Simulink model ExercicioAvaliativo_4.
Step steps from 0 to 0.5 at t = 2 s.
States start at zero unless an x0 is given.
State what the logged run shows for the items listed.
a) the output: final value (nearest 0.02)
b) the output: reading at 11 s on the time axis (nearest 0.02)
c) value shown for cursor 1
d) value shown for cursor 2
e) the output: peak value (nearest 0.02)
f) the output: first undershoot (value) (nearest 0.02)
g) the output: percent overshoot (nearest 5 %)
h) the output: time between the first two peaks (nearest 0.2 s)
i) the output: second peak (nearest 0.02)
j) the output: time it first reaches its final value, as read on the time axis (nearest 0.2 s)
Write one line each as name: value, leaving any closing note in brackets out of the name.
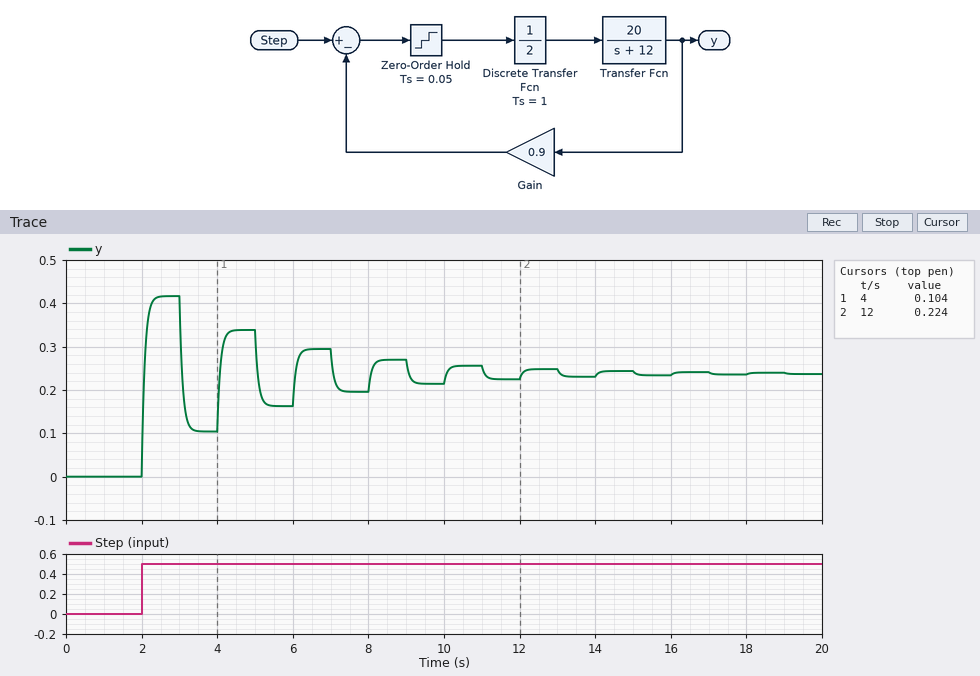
the output: final value: 0.24
the output: reading at 11 s on the time axis: 0.26
value shown for cursor 1: 0.104
value shown for cursor 2: 0.224
the output: peak value: 0.42
the output: first undershoot (value): 0.10
the output: percent overshoot: 75 %
the output: time between the first two peaks: 2.0 s
the output: second peak: 0.34
the output: time it first reaches its final value, as read on the time axis: 2.0 s
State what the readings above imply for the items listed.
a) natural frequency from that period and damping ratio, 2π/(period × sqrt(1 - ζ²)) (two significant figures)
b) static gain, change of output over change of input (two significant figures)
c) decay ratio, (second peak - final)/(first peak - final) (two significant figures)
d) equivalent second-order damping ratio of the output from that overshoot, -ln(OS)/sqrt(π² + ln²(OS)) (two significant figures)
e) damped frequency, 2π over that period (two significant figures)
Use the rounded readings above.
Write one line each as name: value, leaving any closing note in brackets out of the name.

natural frequency from that period and damping ratio, 2π/(period × sqrt(1 - ζ²)): 3.2 rad/s
static gain, change of output over change of input: 0.48
decay ratio, (second peak - final)/(first peak - final): 0.56
equivalent second-order damping ratio of the output from that overshoot, -ln(OS)/sqrt(π² + ln²(OS)): 0.091
damped frequency, 2π over that period: 3.1 rad/s
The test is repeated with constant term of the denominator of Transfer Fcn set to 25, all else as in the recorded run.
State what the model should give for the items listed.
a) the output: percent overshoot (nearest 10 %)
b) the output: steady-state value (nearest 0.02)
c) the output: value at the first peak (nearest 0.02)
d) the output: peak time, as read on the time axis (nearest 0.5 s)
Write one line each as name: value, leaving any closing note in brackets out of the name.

the output: percent overshoot: 40 %
the output: steady-state value: 0.14
the output: value at the first peak: 0.20
the output: peak time, as read on the time axis: 3.0 s
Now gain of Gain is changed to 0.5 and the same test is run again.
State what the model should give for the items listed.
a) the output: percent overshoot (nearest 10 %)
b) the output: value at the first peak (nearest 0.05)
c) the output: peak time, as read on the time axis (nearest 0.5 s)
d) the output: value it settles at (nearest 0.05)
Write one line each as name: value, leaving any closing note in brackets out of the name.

the output: percent overshoot: 40 %
the output: value at the first peak: 0.40
the output: peak time, as read on the time axis: 3.0 s
the output: value it settles at: 0.30
